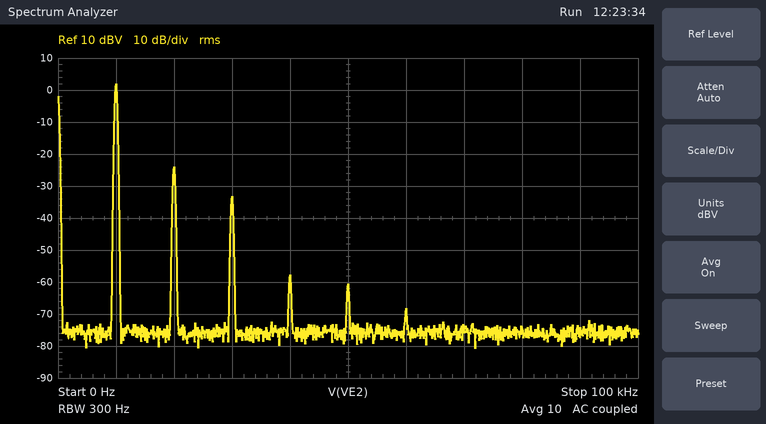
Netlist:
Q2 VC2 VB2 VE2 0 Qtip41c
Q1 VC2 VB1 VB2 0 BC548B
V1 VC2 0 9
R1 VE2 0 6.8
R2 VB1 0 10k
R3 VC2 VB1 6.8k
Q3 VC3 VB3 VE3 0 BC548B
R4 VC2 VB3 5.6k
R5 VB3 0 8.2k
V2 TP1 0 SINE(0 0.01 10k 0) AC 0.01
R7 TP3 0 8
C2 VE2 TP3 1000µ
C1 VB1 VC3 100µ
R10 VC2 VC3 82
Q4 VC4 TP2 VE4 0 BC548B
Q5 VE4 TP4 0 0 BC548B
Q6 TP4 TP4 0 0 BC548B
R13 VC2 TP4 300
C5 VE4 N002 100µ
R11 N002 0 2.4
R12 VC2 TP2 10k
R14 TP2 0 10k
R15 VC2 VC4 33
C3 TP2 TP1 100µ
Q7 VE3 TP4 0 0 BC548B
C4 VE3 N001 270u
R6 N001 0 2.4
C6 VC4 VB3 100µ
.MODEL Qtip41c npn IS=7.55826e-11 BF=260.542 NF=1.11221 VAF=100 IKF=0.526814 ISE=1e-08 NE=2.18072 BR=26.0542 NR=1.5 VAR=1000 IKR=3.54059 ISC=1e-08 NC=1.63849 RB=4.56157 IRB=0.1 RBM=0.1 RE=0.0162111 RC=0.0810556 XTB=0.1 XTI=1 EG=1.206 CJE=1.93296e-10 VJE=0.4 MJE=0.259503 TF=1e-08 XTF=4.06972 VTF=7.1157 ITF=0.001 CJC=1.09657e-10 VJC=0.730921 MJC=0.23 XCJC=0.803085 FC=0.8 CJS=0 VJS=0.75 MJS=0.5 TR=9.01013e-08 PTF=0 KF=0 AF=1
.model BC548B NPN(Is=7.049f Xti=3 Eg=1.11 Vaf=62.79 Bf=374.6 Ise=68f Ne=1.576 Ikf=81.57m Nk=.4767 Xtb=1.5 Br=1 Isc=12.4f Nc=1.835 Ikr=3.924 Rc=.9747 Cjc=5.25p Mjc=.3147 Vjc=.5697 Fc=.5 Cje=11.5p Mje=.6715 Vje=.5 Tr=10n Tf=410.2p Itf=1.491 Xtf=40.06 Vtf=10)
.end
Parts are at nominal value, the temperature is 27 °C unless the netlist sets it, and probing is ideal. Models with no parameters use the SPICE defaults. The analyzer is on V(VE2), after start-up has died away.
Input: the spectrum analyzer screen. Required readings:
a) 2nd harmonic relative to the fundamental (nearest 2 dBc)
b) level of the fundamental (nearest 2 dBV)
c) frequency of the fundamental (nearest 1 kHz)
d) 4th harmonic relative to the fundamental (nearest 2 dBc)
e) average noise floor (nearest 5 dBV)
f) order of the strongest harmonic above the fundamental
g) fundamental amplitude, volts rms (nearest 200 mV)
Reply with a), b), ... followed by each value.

a) -26 dBc
b) 2 dBV
c) 10 kHz
d) -60 dBc
e) -75 dBV
f) 2
g) 1.2 V
